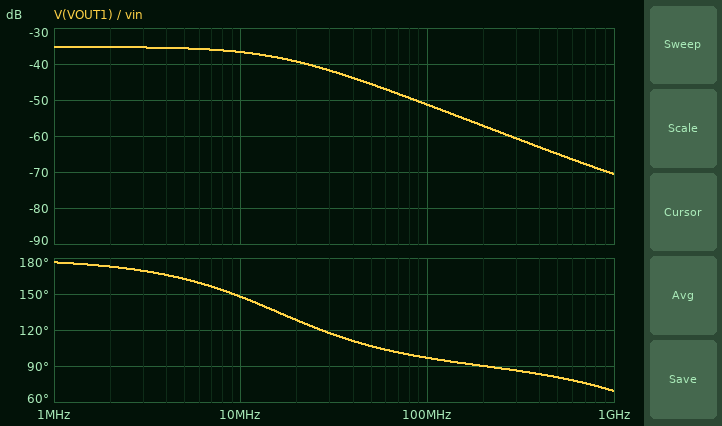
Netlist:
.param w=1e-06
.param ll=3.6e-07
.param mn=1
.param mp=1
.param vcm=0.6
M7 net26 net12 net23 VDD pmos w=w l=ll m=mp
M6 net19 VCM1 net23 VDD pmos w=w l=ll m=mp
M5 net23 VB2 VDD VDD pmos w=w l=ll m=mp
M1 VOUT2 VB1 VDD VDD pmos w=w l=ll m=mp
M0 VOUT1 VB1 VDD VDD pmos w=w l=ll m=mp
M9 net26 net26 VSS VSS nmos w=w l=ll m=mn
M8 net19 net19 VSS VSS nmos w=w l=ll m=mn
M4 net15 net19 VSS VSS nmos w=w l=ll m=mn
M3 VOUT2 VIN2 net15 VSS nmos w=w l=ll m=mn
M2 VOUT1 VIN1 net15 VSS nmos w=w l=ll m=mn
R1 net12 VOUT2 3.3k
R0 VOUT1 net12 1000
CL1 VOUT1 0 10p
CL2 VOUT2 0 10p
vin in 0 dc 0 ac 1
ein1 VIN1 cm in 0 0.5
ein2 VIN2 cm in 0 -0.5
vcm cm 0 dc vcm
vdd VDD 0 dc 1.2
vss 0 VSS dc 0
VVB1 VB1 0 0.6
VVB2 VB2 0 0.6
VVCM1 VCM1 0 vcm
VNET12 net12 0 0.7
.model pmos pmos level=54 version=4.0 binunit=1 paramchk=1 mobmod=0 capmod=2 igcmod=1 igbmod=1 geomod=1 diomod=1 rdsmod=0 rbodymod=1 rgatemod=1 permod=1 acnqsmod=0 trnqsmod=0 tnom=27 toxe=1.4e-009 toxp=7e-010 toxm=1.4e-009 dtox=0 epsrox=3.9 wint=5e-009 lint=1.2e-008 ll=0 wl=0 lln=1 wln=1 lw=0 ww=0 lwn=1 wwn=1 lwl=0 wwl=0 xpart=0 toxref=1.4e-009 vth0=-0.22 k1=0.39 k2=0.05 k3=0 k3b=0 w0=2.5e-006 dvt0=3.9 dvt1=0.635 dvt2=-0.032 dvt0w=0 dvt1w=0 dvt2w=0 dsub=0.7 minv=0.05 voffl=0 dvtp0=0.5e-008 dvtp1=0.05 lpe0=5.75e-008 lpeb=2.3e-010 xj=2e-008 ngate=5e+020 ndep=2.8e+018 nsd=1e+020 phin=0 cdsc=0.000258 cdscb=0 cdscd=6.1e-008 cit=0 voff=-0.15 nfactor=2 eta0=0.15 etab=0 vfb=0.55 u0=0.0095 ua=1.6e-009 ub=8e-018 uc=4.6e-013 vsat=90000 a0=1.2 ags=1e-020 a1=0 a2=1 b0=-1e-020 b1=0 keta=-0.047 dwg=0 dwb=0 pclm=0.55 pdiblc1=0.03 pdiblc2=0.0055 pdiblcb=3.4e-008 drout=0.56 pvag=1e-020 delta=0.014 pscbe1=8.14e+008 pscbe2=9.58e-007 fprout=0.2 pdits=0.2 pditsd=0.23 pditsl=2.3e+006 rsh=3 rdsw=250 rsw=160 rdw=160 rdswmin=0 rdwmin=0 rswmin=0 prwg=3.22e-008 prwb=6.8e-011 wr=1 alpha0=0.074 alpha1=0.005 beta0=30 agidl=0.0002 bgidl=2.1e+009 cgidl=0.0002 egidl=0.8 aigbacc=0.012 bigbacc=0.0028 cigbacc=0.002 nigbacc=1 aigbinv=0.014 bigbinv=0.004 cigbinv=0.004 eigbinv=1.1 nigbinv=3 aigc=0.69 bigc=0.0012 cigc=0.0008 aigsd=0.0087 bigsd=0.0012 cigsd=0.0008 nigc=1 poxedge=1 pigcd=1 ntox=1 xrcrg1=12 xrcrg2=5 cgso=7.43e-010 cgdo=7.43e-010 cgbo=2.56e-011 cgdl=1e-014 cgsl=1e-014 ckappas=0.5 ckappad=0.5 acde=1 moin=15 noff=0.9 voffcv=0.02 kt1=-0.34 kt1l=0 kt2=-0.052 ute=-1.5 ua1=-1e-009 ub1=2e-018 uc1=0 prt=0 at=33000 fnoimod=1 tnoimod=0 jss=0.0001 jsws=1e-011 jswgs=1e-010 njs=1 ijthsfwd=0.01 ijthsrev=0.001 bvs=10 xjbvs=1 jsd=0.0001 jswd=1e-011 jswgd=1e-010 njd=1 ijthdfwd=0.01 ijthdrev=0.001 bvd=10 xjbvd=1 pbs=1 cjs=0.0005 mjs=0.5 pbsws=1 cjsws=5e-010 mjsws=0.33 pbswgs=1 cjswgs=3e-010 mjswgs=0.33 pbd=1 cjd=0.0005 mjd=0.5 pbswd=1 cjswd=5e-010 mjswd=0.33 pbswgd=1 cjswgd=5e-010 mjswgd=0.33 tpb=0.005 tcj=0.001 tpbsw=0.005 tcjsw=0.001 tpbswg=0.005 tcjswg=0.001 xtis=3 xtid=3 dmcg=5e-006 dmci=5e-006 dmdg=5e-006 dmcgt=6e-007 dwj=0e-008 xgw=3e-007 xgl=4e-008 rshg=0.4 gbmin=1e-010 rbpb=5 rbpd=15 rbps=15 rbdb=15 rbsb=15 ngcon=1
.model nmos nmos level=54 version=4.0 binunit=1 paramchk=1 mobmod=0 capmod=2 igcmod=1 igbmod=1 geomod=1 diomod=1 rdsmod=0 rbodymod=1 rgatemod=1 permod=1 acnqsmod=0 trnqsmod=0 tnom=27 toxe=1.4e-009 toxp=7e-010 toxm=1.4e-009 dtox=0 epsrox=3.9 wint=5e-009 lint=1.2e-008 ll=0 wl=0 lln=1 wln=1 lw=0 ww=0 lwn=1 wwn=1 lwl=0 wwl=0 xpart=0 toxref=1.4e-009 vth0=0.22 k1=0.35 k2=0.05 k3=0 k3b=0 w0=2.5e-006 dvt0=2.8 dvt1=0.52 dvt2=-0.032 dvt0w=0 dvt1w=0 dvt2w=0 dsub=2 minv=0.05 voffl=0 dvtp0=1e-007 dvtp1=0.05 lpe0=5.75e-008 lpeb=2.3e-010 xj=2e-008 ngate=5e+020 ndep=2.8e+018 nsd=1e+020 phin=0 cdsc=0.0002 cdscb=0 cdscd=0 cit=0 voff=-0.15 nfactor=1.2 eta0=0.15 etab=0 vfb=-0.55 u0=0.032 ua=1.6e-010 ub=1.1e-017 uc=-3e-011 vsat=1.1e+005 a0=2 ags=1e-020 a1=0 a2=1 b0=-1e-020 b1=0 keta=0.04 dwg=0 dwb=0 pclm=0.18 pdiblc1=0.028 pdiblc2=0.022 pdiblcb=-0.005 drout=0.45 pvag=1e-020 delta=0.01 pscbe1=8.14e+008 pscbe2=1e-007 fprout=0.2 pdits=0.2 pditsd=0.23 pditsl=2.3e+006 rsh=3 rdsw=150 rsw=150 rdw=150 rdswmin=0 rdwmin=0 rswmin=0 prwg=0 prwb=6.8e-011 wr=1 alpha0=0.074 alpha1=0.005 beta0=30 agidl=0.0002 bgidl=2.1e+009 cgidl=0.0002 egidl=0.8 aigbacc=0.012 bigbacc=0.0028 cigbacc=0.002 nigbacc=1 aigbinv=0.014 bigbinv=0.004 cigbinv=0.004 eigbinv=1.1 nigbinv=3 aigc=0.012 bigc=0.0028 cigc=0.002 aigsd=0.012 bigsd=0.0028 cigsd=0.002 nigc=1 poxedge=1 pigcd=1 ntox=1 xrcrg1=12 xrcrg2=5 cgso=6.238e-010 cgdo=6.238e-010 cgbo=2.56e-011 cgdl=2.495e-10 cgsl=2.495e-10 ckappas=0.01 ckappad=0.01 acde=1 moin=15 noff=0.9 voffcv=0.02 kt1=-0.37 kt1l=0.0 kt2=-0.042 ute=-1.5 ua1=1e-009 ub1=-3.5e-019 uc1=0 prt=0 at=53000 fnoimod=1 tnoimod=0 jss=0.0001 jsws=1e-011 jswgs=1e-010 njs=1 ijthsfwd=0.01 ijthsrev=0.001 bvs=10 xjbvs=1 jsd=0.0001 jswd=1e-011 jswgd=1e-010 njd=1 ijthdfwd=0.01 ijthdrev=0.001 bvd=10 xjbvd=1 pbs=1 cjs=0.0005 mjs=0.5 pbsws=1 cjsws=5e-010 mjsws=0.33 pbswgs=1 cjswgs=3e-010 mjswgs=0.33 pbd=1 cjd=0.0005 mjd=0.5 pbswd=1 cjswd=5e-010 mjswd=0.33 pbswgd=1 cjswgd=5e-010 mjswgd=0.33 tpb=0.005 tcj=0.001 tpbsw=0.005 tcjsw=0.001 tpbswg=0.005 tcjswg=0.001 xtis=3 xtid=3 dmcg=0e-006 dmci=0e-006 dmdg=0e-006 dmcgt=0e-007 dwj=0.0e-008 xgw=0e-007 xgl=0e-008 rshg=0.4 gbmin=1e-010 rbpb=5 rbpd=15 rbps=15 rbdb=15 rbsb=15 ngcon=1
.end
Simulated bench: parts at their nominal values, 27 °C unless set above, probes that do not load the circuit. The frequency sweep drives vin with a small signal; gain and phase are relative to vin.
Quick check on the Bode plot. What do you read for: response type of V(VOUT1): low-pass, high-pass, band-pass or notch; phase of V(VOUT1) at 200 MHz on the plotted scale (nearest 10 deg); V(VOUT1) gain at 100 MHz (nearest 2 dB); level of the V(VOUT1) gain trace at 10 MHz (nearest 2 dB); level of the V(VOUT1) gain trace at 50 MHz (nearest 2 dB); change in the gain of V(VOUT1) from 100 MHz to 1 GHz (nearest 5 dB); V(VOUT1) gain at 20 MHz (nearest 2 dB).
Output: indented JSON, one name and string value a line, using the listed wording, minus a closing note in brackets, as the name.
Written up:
{
  "response type of V(VOUT1): low-pass, high-pass, band-pass or notch": "low-pass",
  "phase of V(VOUT1) at 200 MHz on the plotted scale": "90 deg",
  "V(VOUT1) gain at 100 MHz": "-52 dB",
  "level of the V(VOUT1) gain trace at 10 MHz": "-36 dB",
  "level of the V(VOUT1) gain trace at 50 MHz": "-46 dB",
  "change in the gain of V(VOUT1) from 100 MHz to 1 GHz": "-20 dB",
  "V(VOUT1) gain at 20 MHz": "-40 dB"
}
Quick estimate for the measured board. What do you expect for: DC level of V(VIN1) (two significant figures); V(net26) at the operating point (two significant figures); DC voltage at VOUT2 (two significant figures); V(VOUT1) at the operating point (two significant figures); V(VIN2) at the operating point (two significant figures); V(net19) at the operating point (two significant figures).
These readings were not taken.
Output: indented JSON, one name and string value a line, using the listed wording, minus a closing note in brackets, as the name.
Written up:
{
  "DC level of V(VIN1)": "600 mV",
  "V(net26) at the operating point": "280 mV",
  "DC voltage at VOUT2": "730 mV",
  "V(VOUT1) at the operating point": "710 mV",
  "V(VIN2) at the operating point": "600 mV",
  "V(net19) at the operating point": "340 mV"
}
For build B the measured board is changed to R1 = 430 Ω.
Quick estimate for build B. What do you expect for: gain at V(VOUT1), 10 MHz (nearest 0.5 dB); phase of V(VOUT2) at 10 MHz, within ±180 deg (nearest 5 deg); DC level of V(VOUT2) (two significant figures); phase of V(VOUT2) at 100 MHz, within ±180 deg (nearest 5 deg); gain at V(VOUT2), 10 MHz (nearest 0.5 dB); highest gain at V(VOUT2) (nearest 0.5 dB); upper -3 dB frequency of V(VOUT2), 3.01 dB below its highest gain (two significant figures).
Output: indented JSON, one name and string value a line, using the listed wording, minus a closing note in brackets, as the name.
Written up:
{
  "gain at V(VOUT1), 10 MHz": "-36.5 dB",
  "phase of V(VOUT2) at 10 MHz, within ±180 deg": "-15 deg",
  "DC level of V(VOUT2)": "700 mV",
  "phase of V(VOUT2) at 100 MHz, within ±180 deg": "-70 deg",
  "gain at V(VOUT2), 10 MHz": "-43.0 dB",
  "highest gain at V(VOUT2)": "-42.5 dB",
  "upper -3 dB frequency of V(VOUT2), 3.01 dB below its highest gain": "37 MHz"
}
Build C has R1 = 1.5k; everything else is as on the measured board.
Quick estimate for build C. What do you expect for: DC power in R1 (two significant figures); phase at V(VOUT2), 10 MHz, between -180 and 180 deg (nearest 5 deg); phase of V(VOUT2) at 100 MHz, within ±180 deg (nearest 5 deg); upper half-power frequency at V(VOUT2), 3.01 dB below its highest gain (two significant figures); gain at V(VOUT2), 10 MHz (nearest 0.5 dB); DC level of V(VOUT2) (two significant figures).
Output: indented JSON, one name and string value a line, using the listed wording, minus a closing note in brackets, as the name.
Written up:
{
  "DC power in R1": "130 nW",
  "phase at V(VOUT2), 10 MHz, between -180 and 180 deg": "-45 deg",
  "phase of V(VOUT2) at 100 MHz, within ±180 deg": "-85 deg",
  "upper half-power frequency at V(VOUT2), 3.01 dB below its highest gain": "11 MHz",
  "gain at V(VOUT2), 10 MHz": "-34.5 dB",
  "DC level of V(VOUT2)": "710 mV"
}
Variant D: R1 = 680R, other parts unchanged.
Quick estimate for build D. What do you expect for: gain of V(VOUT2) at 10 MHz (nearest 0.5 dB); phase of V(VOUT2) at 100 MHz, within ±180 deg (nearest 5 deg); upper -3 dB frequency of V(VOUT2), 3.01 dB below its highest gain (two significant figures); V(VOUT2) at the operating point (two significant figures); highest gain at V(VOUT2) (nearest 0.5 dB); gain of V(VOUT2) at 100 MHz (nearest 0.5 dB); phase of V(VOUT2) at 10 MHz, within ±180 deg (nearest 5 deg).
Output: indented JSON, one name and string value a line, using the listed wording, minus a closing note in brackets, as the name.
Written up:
{
  "gain of V(VOUT2) at 10 MHz": "-39.5 dB",
  "phase of V(VOUT2) at 100 MHz, within ±180 deg": "-80 deg",
  "upper -3 dB frequency of V(VOUT2), 3.01 dB below its highest gain": "23 MHz",
  "V(VOUT2) at the operating point": "710 mV",
  "highest gain at V(VOUT2)": "-38.5 dB",
  "gain of V(VOUT2) at 100 MHz": "-51.5 dB",
  "phase of V(VOUT2) at 10 MHz, within ±180 deg": "-25 deg"
}
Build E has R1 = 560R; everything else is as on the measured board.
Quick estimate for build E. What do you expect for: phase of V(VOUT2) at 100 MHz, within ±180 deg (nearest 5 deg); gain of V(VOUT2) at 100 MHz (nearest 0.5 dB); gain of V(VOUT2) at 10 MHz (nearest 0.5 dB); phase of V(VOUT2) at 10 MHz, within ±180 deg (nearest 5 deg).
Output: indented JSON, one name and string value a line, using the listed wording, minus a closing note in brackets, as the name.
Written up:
{
  "phase of V(VOUT2) at 100 MHz, within ±180 deg": "-75 deg",
  "gain of V(VOUT2) at 100 MHz": "-51.5 dB",
  "gain of V(VOUT2) at 10 MHz": "-41.0 dB",
  "phase of V(VOUT2) at 10 MHz, within ±180 deg": "-20 deg"
}
